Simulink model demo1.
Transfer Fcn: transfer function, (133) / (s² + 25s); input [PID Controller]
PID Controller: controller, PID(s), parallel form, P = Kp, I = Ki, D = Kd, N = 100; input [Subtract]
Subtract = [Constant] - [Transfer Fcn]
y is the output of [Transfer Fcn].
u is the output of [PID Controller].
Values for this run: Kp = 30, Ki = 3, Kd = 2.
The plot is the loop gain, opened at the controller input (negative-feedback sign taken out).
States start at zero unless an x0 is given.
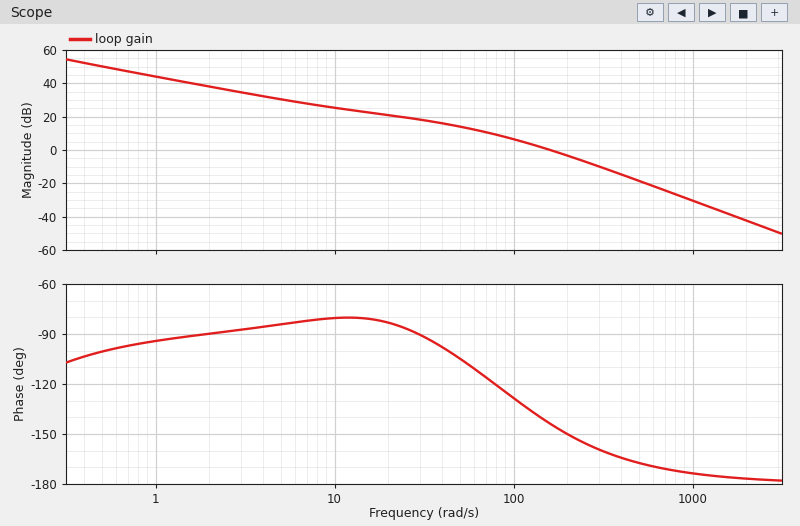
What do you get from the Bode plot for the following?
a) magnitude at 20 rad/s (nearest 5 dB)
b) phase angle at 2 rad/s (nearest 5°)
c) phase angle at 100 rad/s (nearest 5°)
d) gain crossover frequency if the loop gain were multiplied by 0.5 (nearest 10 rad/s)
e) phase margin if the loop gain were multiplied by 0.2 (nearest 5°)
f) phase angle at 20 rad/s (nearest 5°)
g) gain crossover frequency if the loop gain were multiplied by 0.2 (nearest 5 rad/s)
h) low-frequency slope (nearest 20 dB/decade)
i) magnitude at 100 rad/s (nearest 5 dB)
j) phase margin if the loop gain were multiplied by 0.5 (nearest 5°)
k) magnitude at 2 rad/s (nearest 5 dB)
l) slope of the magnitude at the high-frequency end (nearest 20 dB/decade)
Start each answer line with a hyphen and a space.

- 20 dB
- -90°
- -130°
- 100 rad/s
- 75°
- -85°
- 50 rad/s
- -20 dB/decade
- 5 dB
- 50°
- 40 dB
- -40 dB/decade
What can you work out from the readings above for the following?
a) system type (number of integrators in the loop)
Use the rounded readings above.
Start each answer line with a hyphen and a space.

- 1
